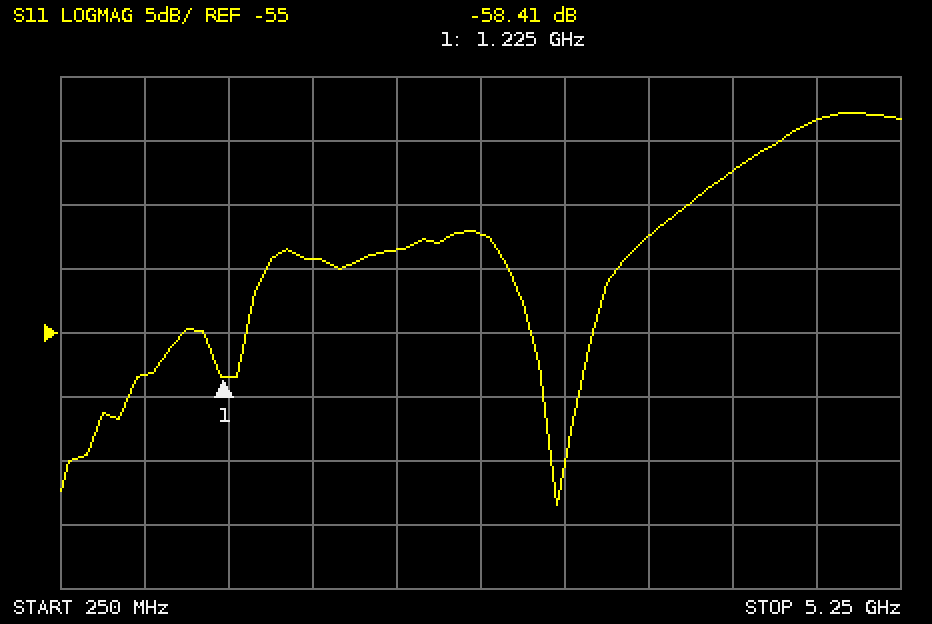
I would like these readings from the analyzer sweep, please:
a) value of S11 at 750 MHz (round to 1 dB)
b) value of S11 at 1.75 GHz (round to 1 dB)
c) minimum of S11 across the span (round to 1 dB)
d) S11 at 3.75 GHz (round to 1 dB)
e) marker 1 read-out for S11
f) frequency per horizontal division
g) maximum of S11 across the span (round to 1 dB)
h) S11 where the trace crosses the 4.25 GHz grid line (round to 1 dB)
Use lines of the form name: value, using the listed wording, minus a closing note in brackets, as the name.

value of S11 at 750 MHz: -58 dB
value of S11 at 1.75 GHz: -49 dB
minimum of S11 across the span: -68 dB
S11 at 3.75 GHz: -47 dB
marker 1 read-out for S11: -58.41 dB
frequency per horizontal division: 500 MHz
maximum of S11 across the span: -38 dB
S11 where the trace crosses the 4.25 GHz grid line: -42 dB
